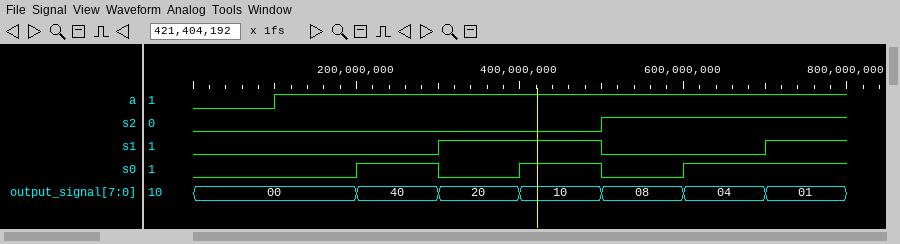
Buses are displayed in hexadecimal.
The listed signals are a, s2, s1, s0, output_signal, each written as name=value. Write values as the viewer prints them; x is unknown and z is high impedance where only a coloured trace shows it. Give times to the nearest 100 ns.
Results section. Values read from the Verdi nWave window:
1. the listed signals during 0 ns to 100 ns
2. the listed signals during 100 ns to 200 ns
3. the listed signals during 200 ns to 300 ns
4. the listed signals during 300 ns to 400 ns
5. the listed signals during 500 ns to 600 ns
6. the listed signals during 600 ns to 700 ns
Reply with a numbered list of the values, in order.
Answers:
1. a=0, s2=0, s1=0, s0=0, output_signal=00
2. a=1, s2=0, s1=0, s0=0, output_signal=00
3. a=1, s2=0, s1=0, s0=1, output_signal=40
4. a=1, s2=0, s1=1, s0=0, output_signal=20
5. a=1, s2=1, s1=0, s0=0, output_signal=08
6. a=1, s2=1, s1=0, s0=1, output_signal=04
